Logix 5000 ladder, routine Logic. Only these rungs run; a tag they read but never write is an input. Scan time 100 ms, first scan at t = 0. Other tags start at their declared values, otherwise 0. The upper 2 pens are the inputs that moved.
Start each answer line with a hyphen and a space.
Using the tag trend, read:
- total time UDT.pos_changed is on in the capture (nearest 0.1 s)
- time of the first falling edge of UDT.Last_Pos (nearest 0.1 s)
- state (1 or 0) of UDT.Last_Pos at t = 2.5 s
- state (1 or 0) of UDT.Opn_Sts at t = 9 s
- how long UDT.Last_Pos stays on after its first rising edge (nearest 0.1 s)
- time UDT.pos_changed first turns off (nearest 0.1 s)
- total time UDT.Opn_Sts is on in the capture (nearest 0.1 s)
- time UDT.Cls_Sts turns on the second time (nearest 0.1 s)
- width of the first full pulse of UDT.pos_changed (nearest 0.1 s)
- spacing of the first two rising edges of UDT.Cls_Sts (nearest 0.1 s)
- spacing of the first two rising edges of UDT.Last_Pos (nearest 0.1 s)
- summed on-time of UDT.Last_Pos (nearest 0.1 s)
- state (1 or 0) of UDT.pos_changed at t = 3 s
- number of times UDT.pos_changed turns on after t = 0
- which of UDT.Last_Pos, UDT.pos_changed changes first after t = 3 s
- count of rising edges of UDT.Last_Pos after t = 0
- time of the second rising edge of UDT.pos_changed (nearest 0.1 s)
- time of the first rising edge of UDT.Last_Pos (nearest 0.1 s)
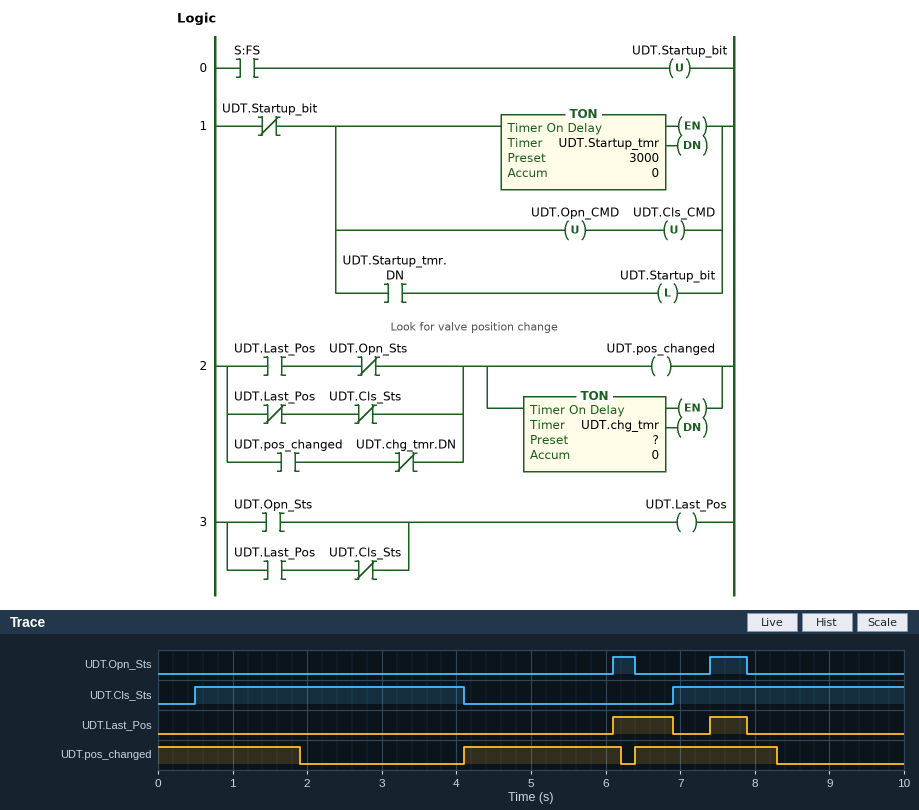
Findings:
- 5.9 s
- 6.9 s
- 0
- 0
- 0.8 s
- 1.9 s
- 0.8 s
- 6.9 s
- 2.1 s
- 6.4 s
- 1.3 s
- 1.3 s
- 0
- 2
- UDT.pos_changed
- 2
- 6.4 s
- 6.1 s
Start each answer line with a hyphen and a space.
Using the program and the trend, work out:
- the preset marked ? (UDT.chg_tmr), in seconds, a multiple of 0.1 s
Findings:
- 1.8 s
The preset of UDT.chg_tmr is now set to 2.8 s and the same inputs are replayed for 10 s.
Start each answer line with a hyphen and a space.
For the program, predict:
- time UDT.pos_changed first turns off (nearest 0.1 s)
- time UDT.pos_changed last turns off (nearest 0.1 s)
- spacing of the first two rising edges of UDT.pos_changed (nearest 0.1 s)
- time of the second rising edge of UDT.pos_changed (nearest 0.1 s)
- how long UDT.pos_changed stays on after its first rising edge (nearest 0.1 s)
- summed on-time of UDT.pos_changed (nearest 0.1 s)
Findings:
- 2.9 s
- 7.0 s
- 3.8 s
- 7.9 s
- 2.9 s
- 7.9 s
